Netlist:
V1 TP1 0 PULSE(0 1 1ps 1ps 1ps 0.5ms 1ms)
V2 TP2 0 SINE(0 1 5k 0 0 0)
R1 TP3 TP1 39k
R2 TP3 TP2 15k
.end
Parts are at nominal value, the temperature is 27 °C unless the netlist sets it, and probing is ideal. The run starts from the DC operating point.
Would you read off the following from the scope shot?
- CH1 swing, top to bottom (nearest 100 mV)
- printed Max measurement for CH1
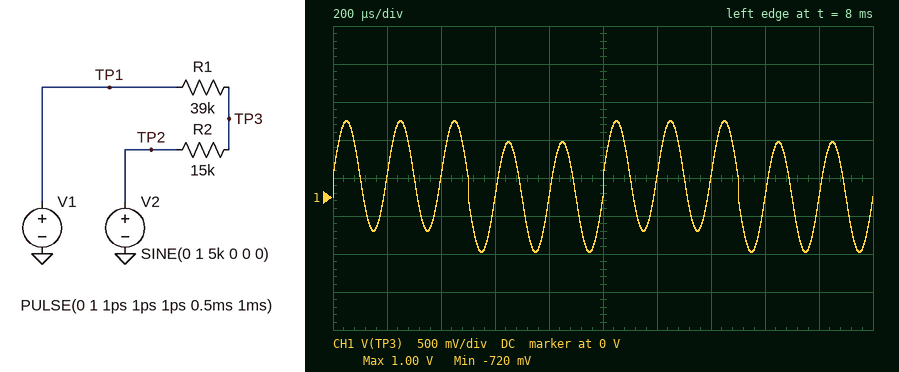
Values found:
1.7 V
1.00 V
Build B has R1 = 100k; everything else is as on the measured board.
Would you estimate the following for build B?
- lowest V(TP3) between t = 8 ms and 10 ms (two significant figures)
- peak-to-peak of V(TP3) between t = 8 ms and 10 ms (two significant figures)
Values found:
-870 mV
1.9 V
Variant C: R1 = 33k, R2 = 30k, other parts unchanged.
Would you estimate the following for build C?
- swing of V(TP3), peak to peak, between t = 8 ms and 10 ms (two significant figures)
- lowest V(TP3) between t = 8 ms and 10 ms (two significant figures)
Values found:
1.5 V
-520 mV
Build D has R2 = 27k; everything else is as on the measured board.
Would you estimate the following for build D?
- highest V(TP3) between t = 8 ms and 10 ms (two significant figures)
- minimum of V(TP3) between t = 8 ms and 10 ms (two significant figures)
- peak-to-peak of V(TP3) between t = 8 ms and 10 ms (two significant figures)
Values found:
1.0 V
-590 mV
1.6 V
